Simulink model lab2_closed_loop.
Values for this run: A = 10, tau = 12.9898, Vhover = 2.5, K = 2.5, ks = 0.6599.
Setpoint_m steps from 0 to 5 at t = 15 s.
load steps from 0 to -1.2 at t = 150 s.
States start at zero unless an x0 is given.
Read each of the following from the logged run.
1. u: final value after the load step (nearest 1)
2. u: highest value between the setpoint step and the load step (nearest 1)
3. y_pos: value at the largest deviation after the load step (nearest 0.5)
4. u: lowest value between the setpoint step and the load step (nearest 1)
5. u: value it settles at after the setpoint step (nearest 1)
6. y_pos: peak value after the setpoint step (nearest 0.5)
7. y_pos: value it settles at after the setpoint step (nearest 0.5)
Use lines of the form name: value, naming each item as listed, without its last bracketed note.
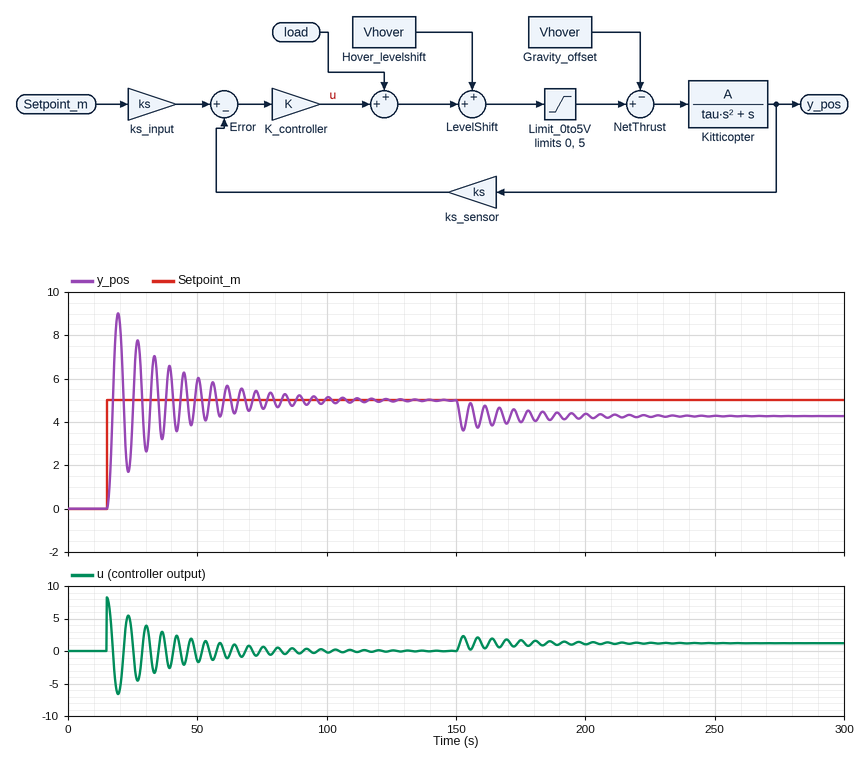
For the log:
u: final value after the load step: 1
u: highest value between the setpoint step and the load step: 8
y_pos: value at the largest deviation after the load step: 3.5
u: lowest value between the setpoint step and the load step: -7
u: value it settles at after the setpoint step: 0
y_pos: peak value after the setpoint step: 9.0
y_pos: value it settles at after the setpoint step: 5.0
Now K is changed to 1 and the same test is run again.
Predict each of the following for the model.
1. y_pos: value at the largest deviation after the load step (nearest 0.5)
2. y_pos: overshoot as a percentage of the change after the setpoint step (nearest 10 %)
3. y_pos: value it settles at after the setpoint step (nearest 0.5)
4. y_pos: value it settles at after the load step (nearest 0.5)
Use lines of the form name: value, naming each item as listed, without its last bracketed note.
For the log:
y_pos: value at the largest deviation after the load step: 1.5
y_pos: overshoot as a percentage of the change after the setpoint step: 80 %
y_pos: value it settles at after the setpoint step: 5.0
y_pos: value it settles at after the load step: 3.0
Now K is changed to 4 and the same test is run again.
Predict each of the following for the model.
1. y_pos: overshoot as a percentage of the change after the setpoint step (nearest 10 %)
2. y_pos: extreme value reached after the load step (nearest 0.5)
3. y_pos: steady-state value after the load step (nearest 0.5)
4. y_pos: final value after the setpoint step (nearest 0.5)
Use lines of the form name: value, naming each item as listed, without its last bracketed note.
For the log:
y_pos: overshoot as a percentage of the change after the setpoint step: 80 %
y_pos: extreme value reached after the load step: 4.0
y_pos: steady-state value after the load step: 4.5
y_pos: final value after the setpoint step: 5.0
